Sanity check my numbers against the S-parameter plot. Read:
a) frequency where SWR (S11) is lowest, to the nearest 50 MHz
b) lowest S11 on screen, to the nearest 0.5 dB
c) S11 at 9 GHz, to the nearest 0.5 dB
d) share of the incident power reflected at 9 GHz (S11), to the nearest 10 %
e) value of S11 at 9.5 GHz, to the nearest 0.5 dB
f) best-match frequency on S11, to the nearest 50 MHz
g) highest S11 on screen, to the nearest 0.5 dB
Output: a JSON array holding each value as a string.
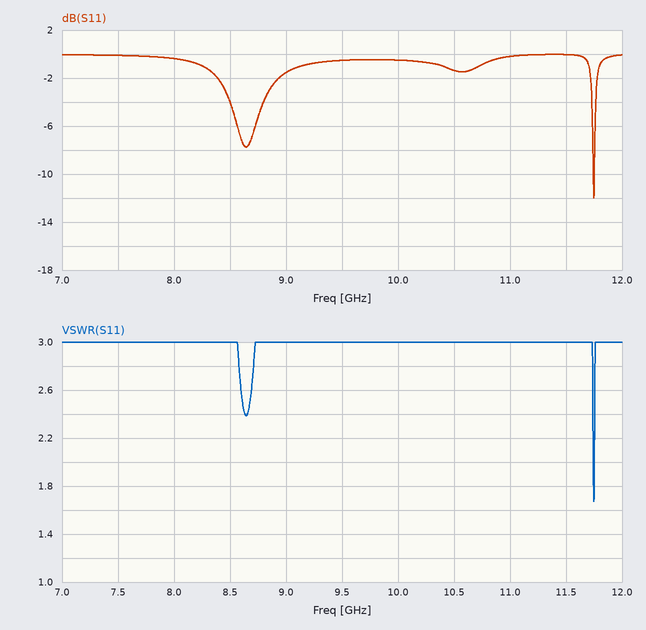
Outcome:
["11.75 GHz", "-12.0 dB", "-1.5 dB", "70 %", "-0.5 dB", "11.75 GHz", "0.0 dB"]
